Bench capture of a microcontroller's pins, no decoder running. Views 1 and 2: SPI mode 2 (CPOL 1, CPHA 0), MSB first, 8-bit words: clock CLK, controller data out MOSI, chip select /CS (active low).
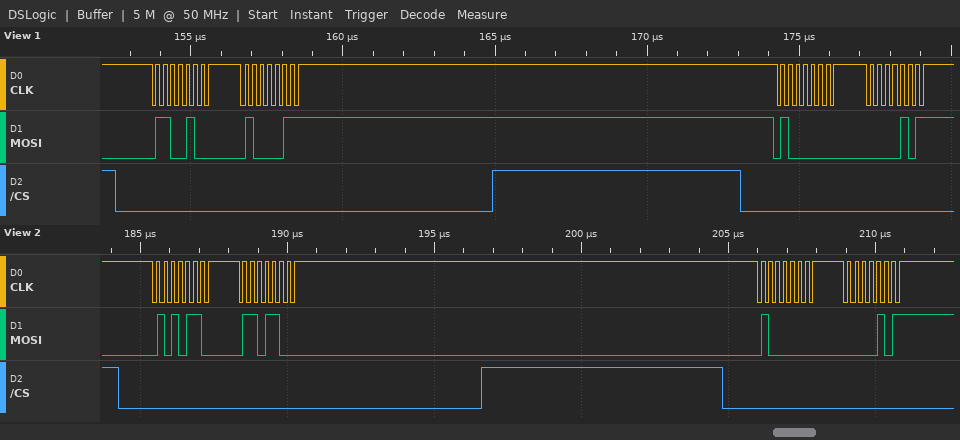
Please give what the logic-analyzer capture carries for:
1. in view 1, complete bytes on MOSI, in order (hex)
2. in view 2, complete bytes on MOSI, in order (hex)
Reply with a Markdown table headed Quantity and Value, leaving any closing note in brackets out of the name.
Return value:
| Quantity | Value |
|---|---|
| in view 1, complete bytes on MOSI, in order | 64 43 40 05 |
| in view 2, complete bytes on MOSI, in order | 56 6C 40 05 |
